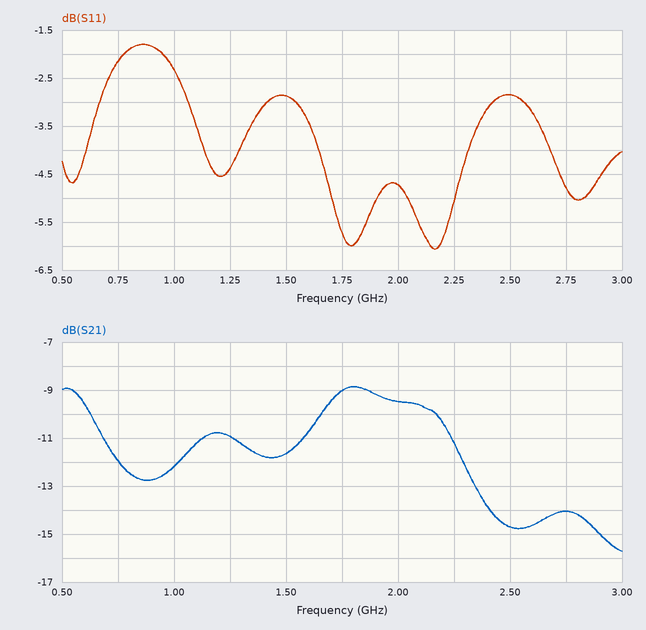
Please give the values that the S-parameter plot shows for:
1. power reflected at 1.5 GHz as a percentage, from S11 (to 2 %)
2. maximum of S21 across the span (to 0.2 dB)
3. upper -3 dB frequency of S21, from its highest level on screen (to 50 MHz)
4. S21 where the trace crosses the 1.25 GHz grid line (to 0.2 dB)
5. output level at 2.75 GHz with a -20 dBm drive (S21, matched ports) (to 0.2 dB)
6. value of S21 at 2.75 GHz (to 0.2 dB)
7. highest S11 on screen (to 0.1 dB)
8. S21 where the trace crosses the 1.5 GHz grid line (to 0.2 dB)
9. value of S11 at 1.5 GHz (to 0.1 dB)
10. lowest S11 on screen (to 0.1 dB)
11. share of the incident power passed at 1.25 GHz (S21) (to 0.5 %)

52 %
-8.8 dB
2.30 GHz
-11.0 dB
-34.0 dBm
-14.0 dB
-1.8 dB
-11.6 dB
-2.9 dB
-6.1 dB
8.0 %
